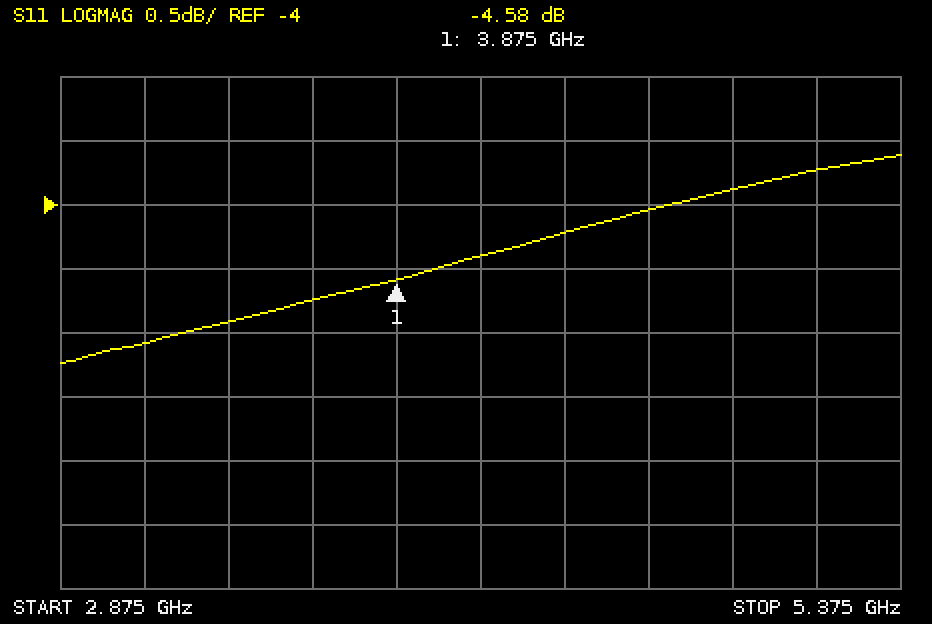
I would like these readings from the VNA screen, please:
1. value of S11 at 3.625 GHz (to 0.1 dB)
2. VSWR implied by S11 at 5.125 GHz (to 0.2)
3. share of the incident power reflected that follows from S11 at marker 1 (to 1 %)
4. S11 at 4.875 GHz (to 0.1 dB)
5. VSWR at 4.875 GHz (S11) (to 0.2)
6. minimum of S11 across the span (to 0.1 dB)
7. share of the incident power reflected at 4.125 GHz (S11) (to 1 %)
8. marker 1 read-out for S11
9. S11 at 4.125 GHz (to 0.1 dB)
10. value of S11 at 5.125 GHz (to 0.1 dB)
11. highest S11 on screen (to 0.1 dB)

-4.7 dB
4.8
35 %
-3.9 dB
4.6
-5.2 dB
36 %
-4.58 dB
-4.4 dB
-3.7 dB
-3.6 dB
